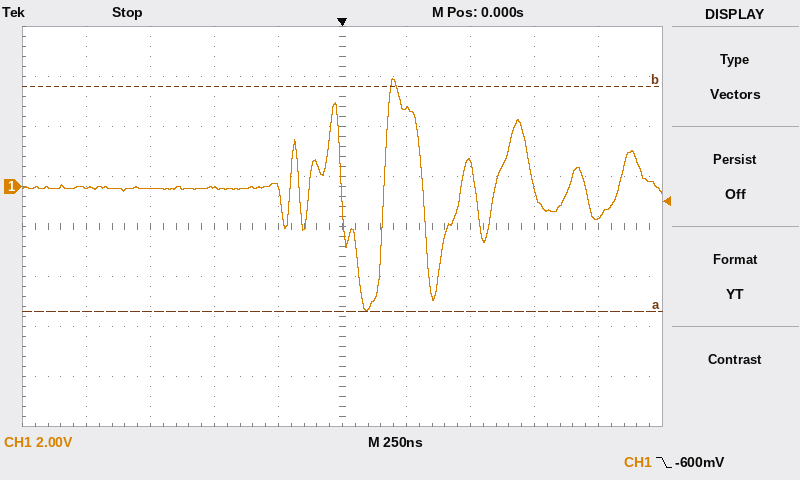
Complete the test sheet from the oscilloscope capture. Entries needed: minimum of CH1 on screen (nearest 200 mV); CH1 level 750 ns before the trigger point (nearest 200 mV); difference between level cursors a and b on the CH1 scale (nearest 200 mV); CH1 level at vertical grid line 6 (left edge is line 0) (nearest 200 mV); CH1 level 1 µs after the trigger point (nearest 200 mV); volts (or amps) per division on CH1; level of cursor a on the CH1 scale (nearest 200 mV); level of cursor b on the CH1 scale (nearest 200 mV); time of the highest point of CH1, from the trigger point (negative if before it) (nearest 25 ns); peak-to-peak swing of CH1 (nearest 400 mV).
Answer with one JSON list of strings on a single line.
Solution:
["-5.0 V", "0.0 V", "9.0 V", "3.2 V", "-1.2 V", "2 V", "-5.0 V", "4.0 V", "+200 ns", "9.2 V"]
